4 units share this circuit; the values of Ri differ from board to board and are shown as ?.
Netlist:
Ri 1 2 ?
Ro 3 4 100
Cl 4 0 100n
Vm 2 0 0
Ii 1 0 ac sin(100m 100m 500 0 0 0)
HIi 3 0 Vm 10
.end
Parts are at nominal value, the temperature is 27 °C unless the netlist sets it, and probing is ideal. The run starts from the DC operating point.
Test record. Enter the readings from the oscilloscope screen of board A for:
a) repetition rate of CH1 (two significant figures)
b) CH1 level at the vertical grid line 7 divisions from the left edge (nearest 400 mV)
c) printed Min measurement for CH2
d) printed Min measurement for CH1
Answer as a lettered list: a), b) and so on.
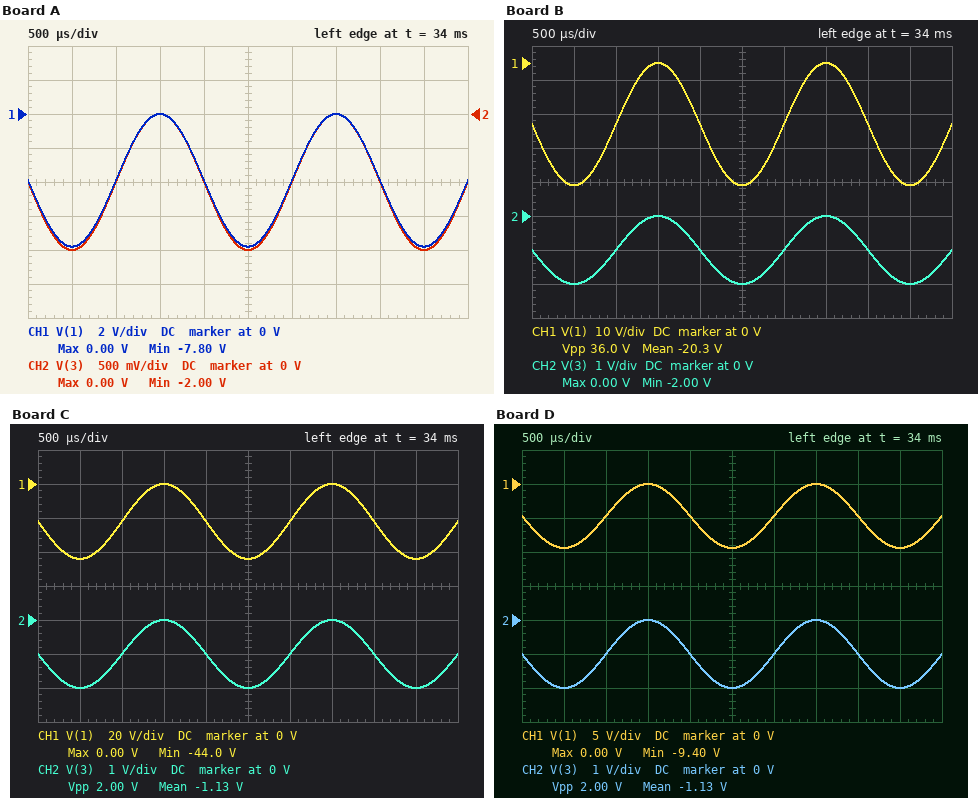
a) 500 Hz
b) 0 V
c) -2.00 V
d) -7.80 V
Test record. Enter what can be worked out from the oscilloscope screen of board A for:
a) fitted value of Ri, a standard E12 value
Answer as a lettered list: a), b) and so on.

a) 39 Ω
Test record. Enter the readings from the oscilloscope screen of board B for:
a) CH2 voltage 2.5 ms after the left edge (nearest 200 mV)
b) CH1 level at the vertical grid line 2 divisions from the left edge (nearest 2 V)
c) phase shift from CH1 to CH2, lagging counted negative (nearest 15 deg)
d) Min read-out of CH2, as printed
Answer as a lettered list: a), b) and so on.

a) -2.0 V
b) -18 V
c) 0 deg
d) -2.00 V
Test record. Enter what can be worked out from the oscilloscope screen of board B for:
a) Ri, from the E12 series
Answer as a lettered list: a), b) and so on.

a) 180 Ω
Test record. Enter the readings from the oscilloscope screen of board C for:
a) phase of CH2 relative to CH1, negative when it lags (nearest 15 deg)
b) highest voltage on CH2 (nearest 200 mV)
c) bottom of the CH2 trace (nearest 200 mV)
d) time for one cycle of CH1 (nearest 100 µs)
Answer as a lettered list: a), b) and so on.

a) 0 deg
b) 0 V
c) -2.0 V
d) 2.0 ms
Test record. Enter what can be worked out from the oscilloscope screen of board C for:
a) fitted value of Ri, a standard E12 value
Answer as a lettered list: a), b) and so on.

a) 220 Ω
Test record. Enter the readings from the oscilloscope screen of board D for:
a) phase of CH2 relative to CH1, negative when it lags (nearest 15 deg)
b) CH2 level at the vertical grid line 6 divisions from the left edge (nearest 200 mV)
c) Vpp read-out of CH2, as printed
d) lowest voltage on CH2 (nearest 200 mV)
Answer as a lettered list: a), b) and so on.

a) 0 deg
b) -1.0 V
c) 2.00 V
d) -2.0 V
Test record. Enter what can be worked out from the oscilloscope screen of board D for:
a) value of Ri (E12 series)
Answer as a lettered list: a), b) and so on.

a) 47 Ω
